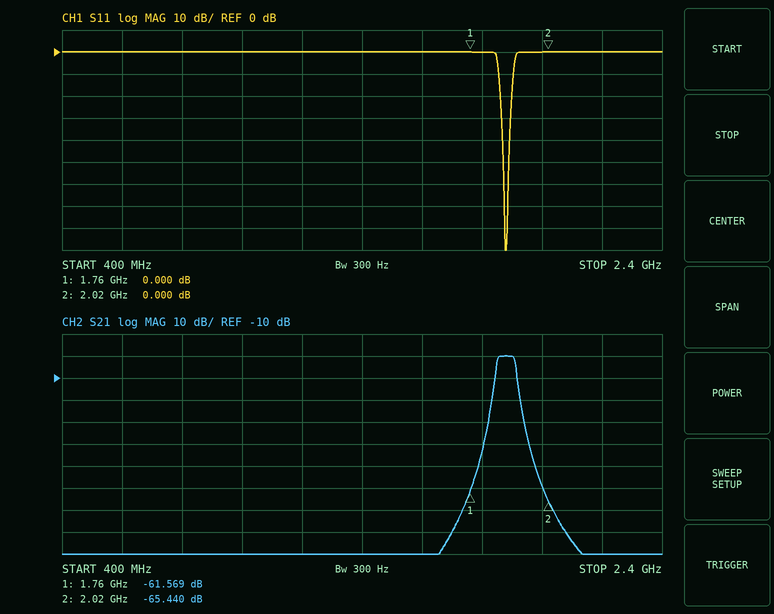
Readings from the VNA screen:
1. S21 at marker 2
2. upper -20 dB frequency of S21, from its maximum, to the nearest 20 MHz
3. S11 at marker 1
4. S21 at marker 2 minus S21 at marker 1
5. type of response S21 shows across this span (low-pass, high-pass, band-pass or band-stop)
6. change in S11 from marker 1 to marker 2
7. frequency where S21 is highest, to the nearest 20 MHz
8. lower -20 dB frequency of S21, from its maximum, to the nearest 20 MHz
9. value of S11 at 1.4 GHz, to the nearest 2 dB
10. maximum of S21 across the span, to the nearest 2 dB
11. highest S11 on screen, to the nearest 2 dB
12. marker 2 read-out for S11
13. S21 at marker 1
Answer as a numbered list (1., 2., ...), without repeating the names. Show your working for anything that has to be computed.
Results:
1. -65.440 dB
2. 1.92 GHz
3. 0.000 dB
4. -65.44 − (-61.569) = -3.871 dB
5. band-pass
6. 0 − (0) = 0.000 dB
7. 1.88 GHz
8. 1.84 GHz
9. 0 dB
10. 0 dB
11. 0 dB
12. 0.000 dB
13. -61.569 dB
